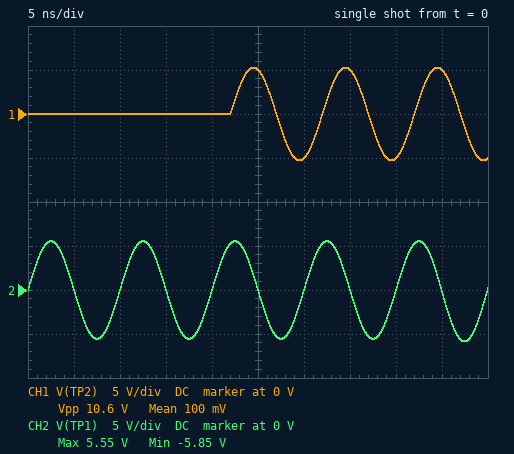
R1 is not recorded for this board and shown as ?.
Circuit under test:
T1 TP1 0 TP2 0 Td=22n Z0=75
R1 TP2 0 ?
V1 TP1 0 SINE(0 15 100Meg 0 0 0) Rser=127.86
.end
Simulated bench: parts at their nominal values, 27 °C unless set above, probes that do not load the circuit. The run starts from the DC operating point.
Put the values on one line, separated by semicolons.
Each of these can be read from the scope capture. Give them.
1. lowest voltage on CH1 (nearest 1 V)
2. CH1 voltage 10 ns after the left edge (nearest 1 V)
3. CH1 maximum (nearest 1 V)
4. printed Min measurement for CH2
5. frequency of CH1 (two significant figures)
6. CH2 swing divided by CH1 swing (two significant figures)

-5 V; 0 V; 5 V; -5.85 V; 100 MHz; 1.1
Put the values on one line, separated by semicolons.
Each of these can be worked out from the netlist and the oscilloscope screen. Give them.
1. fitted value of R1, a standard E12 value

68 Ω
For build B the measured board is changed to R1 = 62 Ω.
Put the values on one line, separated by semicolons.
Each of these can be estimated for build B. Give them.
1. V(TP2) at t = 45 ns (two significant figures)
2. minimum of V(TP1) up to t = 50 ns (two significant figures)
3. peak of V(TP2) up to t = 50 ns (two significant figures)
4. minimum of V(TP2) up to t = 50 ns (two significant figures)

4.8 V; -6.1 V; 5.0 V; -5.0 V
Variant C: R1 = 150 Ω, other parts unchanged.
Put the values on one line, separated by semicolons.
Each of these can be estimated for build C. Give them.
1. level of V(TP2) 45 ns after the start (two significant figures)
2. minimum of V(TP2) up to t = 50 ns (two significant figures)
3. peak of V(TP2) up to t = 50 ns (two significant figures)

7.0 V; -7.4 V; 7.4 V
